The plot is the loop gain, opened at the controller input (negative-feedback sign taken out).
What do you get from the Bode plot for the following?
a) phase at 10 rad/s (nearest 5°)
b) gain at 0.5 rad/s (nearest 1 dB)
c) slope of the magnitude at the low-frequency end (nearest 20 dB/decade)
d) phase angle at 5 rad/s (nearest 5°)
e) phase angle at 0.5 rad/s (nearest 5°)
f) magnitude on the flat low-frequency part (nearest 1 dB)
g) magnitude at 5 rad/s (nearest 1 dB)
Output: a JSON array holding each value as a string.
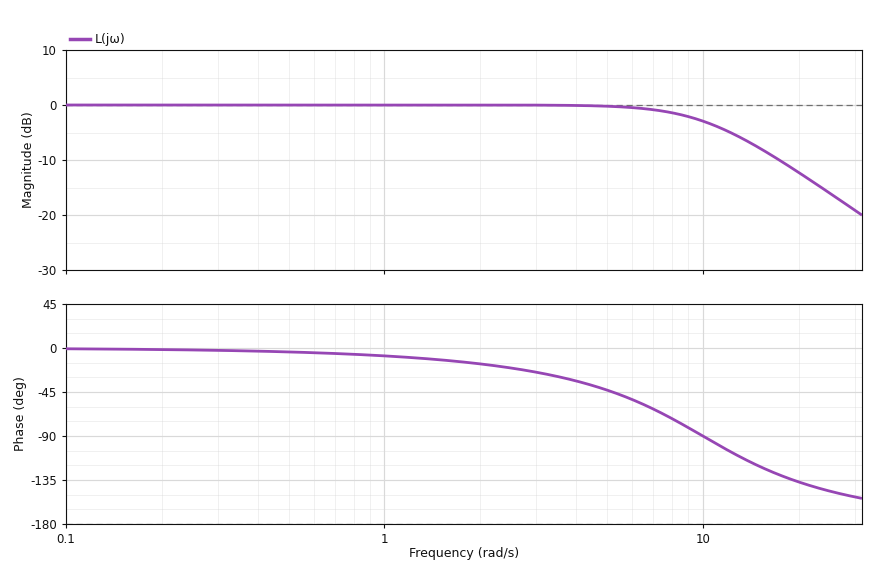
["-90°", "0 dB", "0 dB/decade", "-45°", "-5°", "0 dB", "0 dB"]
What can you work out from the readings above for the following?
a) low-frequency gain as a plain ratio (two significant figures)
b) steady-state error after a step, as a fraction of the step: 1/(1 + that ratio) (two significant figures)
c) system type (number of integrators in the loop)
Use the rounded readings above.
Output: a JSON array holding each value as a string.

["1.0", "0.50", "0"]
